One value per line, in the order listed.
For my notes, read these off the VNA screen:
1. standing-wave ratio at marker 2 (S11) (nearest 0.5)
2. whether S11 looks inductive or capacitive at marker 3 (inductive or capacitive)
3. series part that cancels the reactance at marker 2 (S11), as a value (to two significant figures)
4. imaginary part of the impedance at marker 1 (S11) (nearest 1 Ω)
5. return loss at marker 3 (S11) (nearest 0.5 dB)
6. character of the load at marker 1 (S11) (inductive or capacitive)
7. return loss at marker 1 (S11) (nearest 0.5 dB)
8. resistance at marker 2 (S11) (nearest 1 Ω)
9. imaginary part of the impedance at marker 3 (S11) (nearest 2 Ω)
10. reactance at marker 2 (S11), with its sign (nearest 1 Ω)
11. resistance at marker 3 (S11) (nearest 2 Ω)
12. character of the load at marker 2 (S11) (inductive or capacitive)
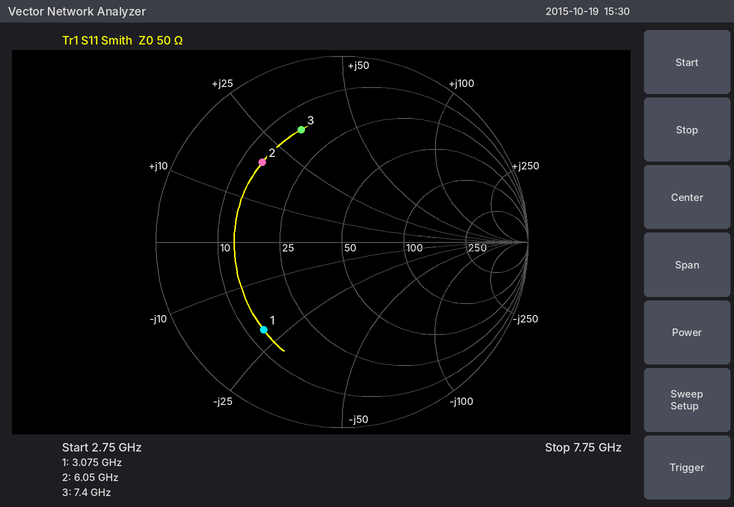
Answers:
4.0
inductive
1.4 pF
-21 Ω
4.0 dB
capacitive
4.0 dB
14 Ω
+32 Ω
+19 Ω
16 Ω
inductive
